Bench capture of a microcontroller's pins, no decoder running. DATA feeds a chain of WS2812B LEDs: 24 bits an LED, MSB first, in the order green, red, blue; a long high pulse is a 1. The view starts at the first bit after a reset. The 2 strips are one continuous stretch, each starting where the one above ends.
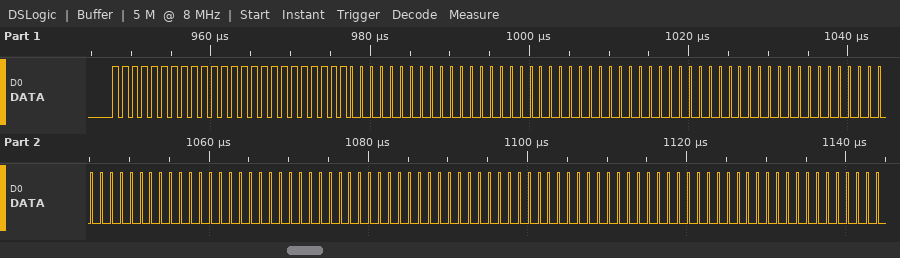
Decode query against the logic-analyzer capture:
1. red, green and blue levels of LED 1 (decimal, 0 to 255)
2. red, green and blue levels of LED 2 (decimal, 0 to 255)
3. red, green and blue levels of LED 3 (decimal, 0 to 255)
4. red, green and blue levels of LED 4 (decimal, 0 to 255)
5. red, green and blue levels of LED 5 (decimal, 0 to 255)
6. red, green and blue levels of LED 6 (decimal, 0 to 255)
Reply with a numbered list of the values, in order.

1. 255, 255, 255
2. 0, 0, 0
3. 0, 0, 0
4. 0, 0, 0
5. 0, 0, 0
6. 0, 0, 0
